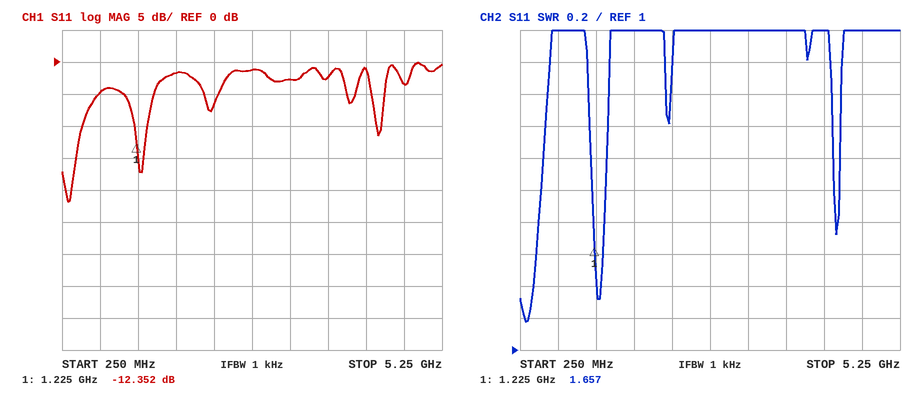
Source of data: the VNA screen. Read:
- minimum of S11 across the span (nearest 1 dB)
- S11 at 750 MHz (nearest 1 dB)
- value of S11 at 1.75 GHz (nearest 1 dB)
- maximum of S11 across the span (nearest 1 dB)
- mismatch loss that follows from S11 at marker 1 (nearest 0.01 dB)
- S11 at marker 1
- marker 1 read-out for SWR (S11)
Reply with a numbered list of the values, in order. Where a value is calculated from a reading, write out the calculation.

1. -22 dB
2. -5 dB
3. -2 dB
4. 0 dB
5. −10 log10(1 − 10^(-12.352/10)) ≈ 0.26 dB
6. -12.352 dB
7. 1.657
